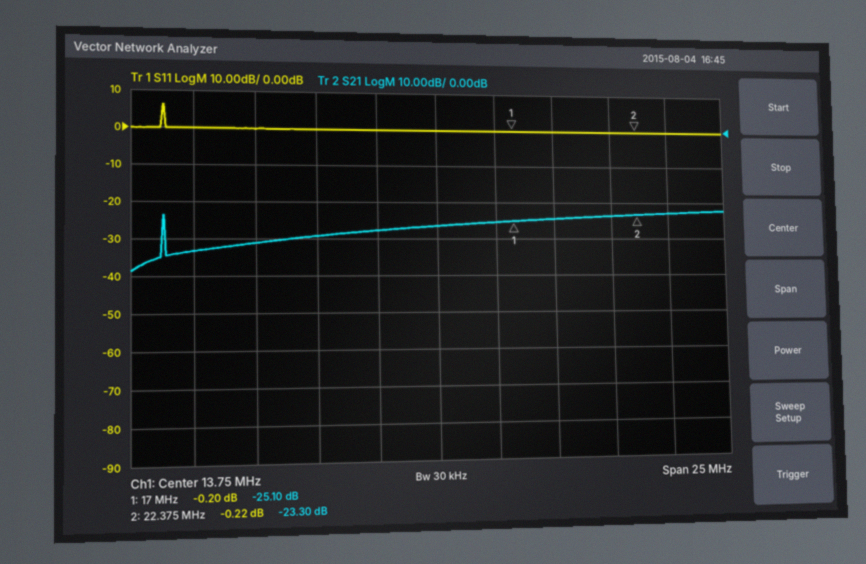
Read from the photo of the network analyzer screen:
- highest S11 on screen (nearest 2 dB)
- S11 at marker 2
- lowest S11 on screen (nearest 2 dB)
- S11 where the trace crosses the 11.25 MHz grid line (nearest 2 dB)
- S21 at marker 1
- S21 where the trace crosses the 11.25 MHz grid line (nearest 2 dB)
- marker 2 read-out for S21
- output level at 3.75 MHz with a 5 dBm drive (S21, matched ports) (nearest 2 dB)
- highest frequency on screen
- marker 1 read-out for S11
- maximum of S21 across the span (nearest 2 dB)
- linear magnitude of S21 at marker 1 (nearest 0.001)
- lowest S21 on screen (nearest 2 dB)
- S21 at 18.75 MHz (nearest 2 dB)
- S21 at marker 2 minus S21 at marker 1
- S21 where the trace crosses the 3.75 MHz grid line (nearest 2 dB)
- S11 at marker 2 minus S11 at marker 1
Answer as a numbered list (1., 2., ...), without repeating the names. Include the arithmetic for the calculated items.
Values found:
1. 6 dB
2. -0.22 dB
3. 0 dB
4. 0 dB
5. -25.10 dB
6. -28 dB
7. -23.30 dB
8. 5 dBm + (-34 dB) = -28 dBm
9. 26.25 MHz
10. -0.20 dB
11. -22 dB
12. 10^(-25.1/20) ≈ 0.056
13. -38 dB
14. -24 dB
15. -23.3 − (-25.1) = 1.80 dB
16. -34 dB
17. -0.22 − (-0.2) = -0.02 dB
